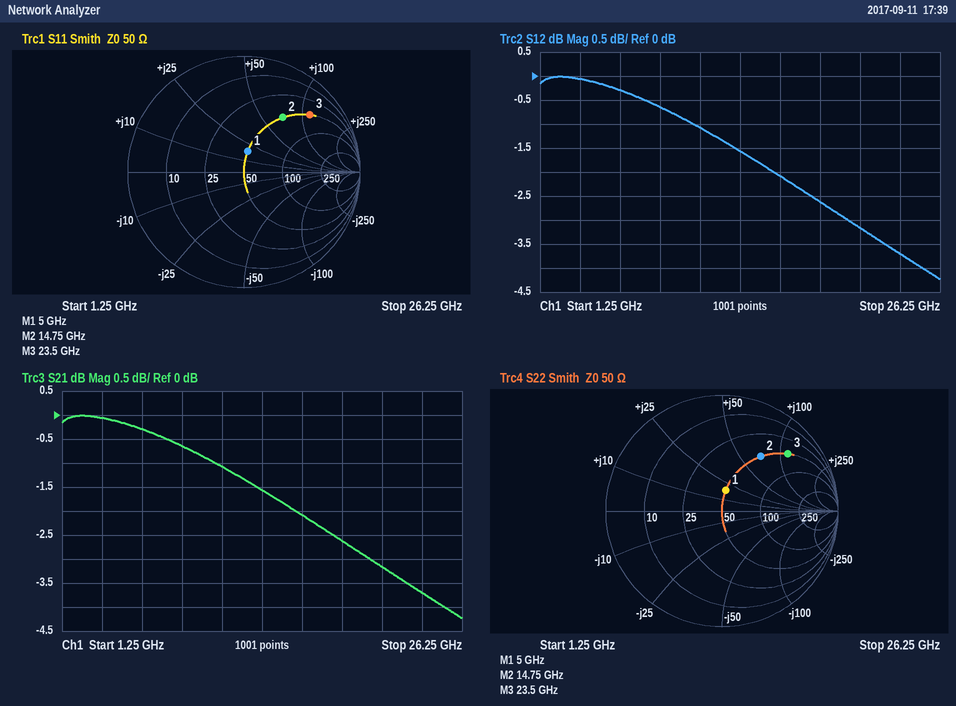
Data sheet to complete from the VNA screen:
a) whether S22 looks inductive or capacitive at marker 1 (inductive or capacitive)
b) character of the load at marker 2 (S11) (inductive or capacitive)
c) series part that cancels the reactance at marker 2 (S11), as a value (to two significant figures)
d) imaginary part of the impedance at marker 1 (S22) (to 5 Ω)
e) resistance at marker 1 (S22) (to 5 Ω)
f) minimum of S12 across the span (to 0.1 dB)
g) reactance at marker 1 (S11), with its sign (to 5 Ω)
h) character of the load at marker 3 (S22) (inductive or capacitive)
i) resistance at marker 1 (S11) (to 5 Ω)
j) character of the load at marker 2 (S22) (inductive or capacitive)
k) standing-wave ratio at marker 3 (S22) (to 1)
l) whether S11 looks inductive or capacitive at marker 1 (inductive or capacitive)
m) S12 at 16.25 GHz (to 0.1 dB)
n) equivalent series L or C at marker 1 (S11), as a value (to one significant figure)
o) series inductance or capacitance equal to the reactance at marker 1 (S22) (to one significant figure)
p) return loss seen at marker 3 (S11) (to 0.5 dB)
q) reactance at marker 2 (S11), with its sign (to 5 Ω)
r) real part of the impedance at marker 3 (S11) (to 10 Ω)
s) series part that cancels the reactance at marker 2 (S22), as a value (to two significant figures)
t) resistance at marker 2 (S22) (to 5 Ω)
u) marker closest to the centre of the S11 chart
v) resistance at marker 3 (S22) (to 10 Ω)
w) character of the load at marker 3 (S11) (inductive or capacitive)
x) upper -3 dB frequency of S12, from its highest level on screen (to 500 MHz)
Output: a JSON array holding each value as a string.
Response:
["inductive", "inductive", "150 fF", "+20 Ω", "50 Ω", "-4.2 dB", "+20 Ω", "inductive", "50 Ω", "inductive", "7", "inductive", "-2.1 dB", "600 pH", "600 pH", "2.5 dB", "+70 Ω", "50 Ω", "150 fF", "50 Ω", "marker 1", "50 Ω", "inductive", "20.5 GHz"]
